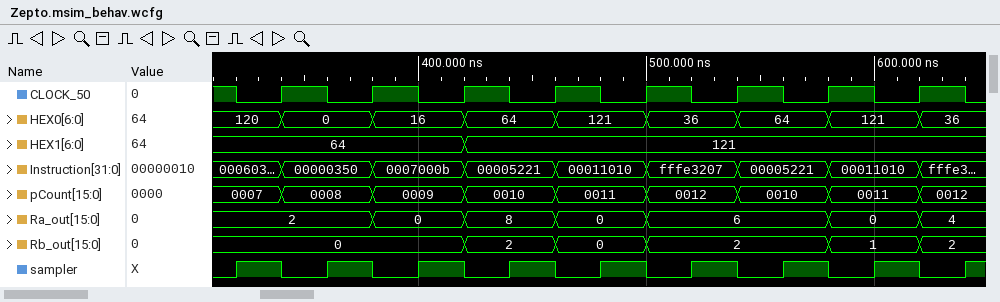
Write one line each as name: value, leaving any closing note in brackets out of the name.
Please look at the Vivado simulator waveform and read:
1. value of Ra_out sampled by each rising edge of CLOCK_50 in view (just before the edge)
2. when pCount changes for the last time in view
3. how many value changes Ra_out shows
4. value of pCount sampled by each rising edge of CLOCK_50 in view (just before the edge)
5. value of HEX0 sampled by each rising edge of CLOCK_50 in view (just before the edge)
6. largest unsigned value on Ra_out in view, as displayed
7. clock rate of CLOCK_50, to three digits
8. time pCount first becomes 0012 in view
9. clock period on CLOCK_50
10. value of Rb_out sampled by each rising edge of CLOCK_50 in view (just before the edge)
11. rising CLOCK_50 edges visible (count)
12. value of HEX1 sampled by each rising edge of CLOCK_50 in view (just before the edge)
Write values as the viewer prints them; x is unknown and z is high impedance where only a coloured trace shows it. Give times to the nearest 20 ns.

value of Ra_out sampled by each rising edge of CLOCK_50 in view: 2, 2, 0, 8, 0, 6, 6, 0
when pCount changes for the last time in view: 620 ns
how many value changes Ra_out shows: 6
value of pCount sampled by each rising edge of CLOCK_50 in view: 0007, 0008, 0009, 0010, 0011, 0012, 0010, 0011
value of HEX0 sampled by each rising edge of CLOCK_50 in view: 120, 0, 16, 64, 121, 36, 64, 121
largest unsigned value on Ra_out in view, as displayed: 8
clock rate of CLOCK_50, to three digits: 25.0 MHz
time pCount first becomes 0012 in view: 500 ns
clock period on CLOCK_50: 40 ns
value of Rb_out sampled by each rising edge of CLOCK_50 in view: 0, 0, 0, 2, 0, 2, 2, 1
rising CLOCK_50 edges visible: 8
value of HEX1 sampled by each rising edge of CLOCK_50 in view: 64, 64, 64, 121, 121, 121, 121, 121
